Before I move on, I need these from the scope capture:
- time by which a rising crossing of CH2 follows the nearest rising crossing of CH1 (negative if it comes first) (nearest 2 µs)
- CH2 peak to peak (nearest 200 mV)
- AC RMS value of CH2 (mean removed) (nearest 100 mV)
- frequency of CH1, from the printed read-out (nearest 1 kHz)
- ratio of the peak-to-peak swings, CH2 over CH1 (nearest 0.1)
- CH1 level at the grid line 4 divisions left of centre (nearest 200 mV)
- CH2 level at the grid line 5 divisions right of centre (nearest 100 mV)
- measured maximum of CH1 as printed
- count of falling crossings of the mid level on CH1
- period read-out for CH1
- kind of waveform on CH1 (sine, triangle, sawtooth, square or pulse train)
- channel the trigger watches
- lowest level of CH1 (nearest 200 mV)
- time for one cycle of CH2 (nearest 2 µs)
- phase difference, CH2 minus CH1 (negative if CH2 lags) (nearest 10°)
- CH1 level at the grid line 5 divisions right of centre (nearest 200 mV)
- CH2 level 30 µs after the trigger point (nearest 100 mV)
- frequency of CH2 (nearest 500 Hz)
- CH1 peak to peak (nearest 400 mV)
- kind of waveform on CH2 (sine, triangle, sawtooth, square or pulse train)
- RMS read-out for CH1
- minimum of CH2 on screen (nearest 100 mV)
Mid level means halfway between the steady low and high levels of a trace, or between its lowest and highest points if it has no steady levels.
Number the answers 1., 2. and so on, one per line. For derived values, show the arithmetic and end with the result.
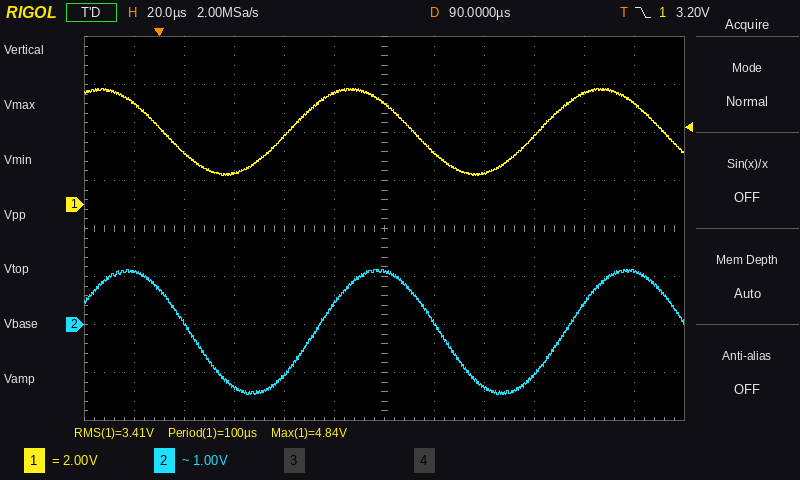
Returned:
1. +10 µs
2. 2.6 V
3. 2.6 V / (2√2) ≈ 919 mV, so 900 mV to the nearest 100 mV
4. 1 / 100 µs ≈ 10 kHz
5. 2.6 V / 3.6 V ≈ 0.7
6. 2.2 V
7. 1.1 V
8. 4.84 V
9. 3
10. 100 µs
11. sine
12. CH1
13. 1.2 V
14. 100 µs
15. −360° × (+10 µs) / 100 µs ≈ -36.0°, so -40° to the nearest 10°
16. 4.2 V
17. -1.3 V
18. 1 / 100 µs ≈ 10.0 kHz
19. 3.6 V
20. sine
21. 3.41 V
22. -1.5 V
